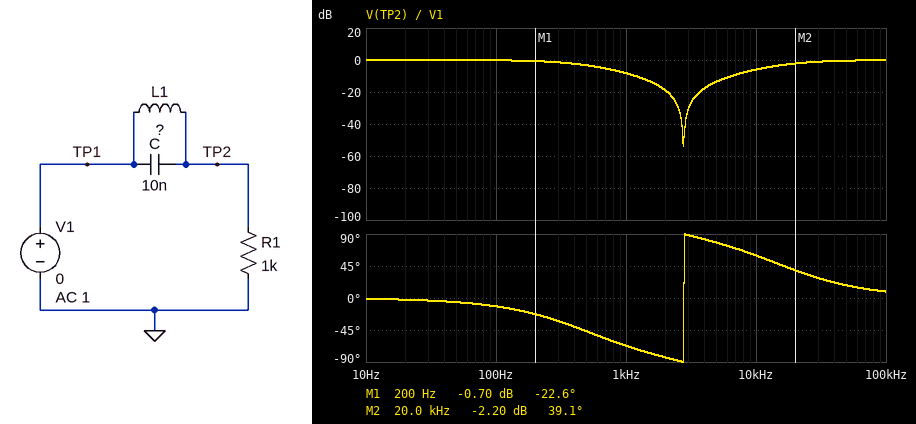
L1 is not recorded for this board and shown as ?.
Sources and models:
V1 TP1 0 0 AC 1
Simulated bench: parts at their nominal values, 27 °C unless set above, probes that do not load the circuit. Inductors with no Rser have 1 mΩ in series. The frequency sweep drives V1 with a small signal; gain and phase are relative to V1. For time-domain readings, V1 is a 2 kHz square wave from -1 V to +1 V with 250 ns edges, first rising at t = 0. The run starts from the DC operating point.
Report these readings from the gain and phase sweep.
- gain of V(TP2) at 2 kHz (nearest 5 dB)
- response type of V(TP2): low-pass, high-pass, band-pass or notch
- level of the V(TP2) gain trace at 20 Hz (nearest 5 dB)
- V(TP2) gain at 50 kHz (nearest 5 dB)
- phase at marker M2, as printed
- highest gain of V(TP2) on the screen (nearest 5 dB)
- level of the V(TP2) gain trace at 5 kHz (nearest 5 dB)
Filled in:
-20 dB
notch
0 dB
0 dB
39.1 deg
0 dB
-15 dB
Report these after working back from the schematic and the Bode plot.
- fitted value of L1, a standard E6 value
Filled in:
330 mH
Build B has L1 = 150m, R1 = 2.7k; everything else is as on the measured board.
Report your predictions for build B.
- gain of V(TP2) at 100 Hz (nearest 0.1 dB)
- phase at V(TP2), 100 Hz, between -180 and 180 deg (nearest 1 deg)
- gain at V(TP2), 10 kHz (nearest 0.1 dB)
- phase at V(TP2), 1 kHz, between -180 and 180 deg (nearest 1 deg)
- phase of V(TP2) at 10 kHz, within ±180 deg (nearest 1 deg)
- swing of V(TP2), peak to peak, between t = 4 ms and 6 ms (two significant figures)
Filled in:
0 dB
-2 deg
-1.8 dB
-20 deg
35 deg
2.1 V
